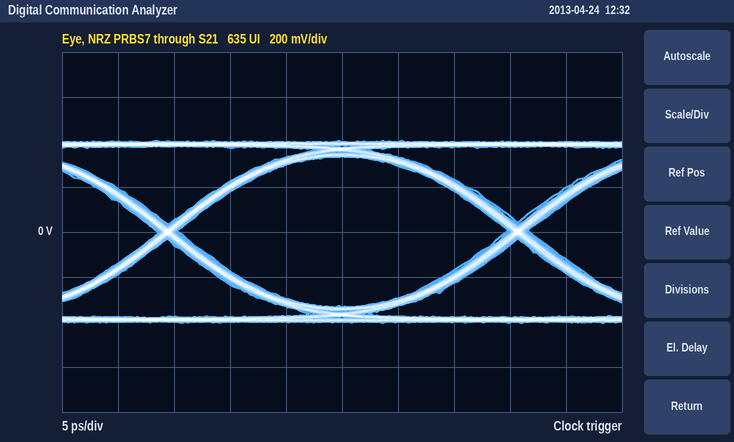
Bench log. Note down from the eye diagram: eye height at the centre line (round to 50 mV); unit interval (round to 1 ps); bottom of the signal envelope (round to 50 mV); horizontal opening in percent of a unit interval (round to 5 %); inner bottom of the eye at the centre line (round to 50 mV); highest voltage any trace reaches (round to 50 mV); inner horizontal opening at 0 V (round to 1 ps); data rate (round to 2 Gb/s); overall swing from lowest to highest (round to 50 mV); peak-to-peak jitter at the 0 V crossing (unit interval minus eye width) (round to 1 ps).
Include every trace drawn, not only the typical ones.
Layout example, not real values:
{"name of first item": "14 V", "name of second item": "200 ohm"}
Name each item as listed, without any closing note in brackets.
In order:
{"eye height at the centre line": "650 mV", "unit interval": "31 ps", "bottom of the signal envelope": "-400 mV", "horizontal opening in percent of a unit interval": "95 %", "inner bottom of the eye at the centre line": "-350 mV", "highest voltage any trace reaches": "400 mV", "inner horizontal opening at 0 V": "29 ps", "data rate": "32 Gb/s", "overall swing from lowest to highest": "800 mV", "peak-to-peak jitter at the 0 V crossing (unit interval minus eye width)": "2 ps"}
